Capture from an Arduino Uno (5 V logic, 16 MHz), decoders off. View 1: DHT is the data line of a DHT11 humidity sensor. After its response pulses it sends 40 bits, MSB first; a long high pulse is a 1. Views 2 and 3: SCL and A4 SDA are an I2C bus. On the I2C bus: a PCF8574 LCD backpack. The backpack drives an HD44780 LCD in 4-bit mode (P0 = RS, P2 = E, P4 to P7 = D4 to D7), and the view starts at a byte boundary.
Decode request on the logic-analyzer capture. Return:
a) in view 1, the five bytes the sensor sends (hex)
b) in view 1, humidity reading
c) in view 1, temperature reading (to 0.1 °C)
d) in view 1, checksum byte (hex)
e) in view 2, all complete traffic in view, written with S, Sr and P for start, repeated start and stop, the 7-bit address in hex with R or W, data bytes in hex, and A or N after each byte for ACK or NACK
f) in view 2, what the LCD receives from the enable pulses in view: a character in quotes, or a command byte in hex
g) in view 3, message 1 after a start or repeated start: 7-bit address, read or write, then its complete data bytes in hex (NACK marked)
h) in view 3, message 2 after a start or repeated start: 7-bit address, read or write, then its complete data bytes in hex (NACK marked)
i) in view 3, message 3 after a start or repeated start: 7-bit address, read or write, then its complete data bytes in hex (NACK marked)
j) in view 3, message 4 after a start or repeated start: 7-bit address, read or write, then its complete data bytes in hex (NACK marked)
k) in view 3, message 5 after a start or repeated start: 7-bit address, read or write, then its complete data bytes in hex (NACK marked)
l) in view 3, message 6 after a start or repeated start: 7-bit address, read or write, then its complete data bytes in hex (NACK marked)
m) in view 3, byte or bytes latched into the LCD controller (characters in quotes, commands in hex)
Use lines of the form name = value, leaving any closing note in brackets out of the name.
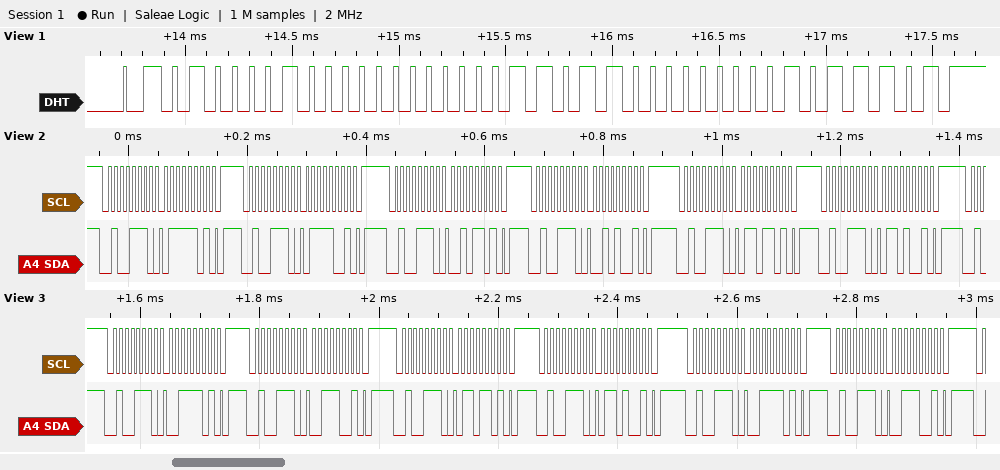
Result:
in view 1, the five bytes the sensor sends = 42 00 1B 00 5D
in view 1, humidity reading = 66 %
in view 1, temperature reading = 27.0 °C
in view 1, checksum byte = 0x5D
in view 2, all complete traffic in view, written with S, Sr and P for start, repeated start and stop, the 7-bit address in hex with R or W, data bytes in hex, and A or N after each byte for ACK or NACK = S 27W A 7D A P S 27W A 79 A P S 27W A 2D A P S 27W A 29 A P S 27W A 6D A P S 27W A 69 A P
in view 2, what the LCD receives from the enable pulses in view: a character in quotes, or a command byte in hex = 'r'
in view 3, message 1 after a start or repeated start: 7-bit address, read or write, then its complete data bytes in hex = 0x27 write: 3D
in view 3, message 2 after a start or repeated start: 7-bit address, read or write, then its complete data bytes in hex = 0x27 write: 39
in view 3, message 3 after a start or repeated start: 7-bit address, read or write, then its complete data bytes in hex = 0x27 write: 6D
in view 3, message 4 after a start or repeated start: 7-bit address, read or write, then its complete data bytes in hex = 0x27 write: 69
in view 3, message 5 after a start or repeated start: 7-bit address, read or write, then its complete data bytes in hex = 0x27 write: 3D
in view 3, message 6 after a start or repeated start: 7-bit address, read or write, then its complete data bytes in hex = 0x27 write: 39
in view 3, byte or bytes latched into the LCD controller = '6'
